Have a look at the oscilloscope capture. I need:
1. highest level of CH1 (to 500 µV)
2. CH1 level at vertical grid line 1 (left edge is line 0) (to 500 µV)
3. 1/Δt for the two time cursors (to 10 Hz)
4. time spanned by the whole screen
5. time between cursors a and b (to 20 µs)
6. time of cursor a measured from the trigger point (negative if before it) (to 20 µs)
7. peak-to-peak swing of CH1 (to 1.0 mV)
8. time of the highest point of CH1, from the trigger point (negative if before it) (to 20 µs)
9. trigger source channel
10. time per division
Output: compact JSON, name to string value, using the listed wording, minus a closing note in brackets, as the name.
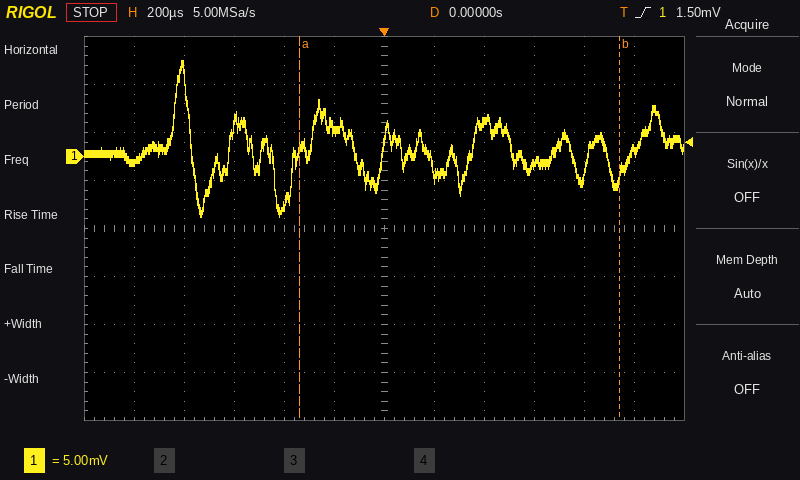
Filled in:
{"highest level of CH1": "10.0 mV", "CH1 level at vertical grid line 1 (left edge is line 0)": "-500 µV", "1/Δt for the two time cursors": "780 Hz", "time spanned by the whole screen": "2.4 ms", "time between cursors a and b": "1.28 ms", "time of cursor a measured from the trigger point (negative if before it)": "-340 µs", "peak-to-peak swing of CH1": "16.0 mV", "time of the highest point of CH1, from the trigger point (negative if before it)": "-800 µs", "trigger source channel": "CH1", "time per division": "200 µs"}
